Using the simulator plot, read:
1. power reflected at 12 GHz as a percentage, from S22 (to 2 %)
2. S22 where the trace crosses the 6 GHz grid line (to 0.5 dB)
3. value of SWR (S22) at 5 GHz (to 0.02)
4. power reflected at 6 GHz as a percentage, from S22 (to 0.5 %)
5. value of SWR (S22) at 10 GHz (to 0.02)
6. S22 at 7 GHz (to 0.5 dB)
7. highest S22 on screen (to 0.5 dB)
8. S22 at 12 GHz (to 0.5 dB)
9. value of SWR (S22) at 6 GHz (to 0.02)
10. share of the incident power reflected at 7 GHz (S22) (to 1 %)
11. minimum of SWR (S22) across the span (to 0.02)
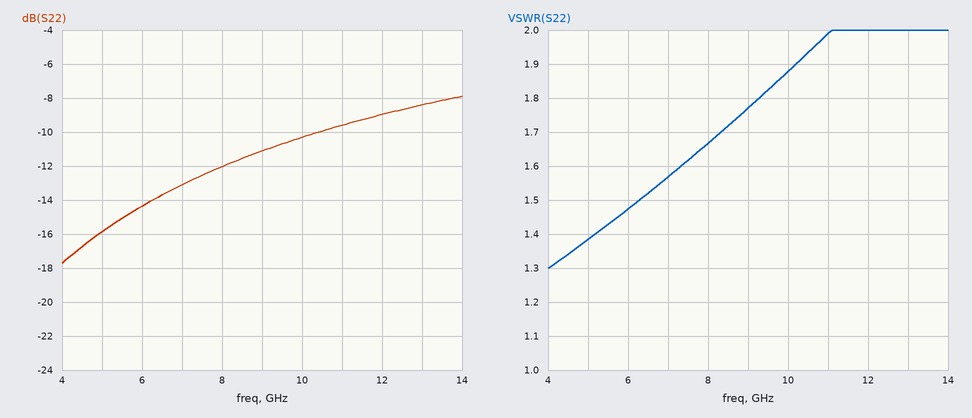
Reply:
12 %
-14.5 dB
1.38
3.5 %
1.88
-13.0 dB
-8.0 dB
-9.0 dB
1.48
5 %
1.30
